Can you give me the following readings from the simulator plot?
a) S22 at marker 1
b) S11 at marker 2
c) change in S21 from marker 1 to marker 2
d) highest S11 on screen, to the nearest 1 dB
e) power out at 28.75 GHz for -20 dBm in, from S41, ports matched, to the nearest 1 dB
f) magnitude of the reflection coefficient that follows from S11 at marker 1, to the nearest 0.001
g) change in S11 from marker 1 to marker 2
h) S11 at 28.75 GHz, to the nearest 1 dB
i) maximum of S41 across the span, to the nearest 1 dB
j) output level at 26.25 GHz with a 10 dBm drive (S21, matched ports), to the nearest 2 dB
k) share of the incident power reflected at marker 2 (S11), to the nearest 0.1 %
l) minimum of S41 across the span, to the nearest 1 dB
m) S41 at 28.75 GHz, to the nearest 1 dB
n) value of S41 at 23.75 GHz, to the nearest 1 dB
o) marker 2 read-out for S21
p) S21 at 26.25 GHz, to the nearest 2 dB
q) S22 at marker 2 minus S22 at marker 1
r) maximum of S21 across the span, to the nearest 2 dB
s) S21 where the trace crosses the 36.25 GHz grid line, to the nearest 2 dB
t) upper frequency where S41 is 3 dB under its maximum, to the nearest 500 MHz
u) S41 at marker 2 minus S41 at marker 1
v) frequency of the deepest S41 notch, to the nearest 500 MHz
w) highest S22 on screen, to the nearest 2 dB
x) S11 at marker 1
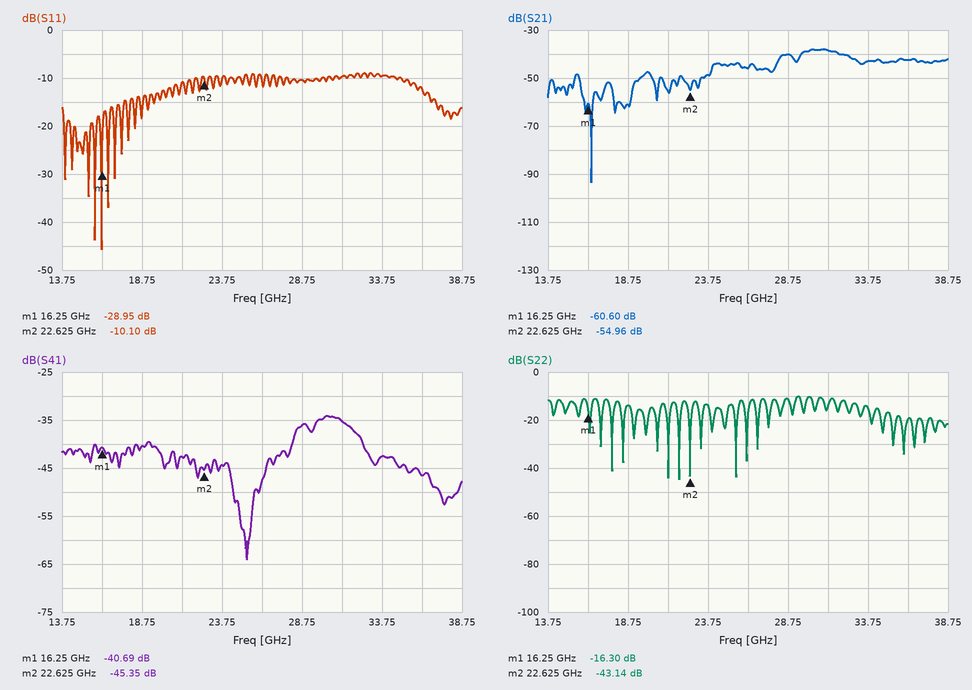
-16.30 dB
-10.10 dB
5.64 dB
-9 dB
-56 dBm
0.036
18.85 dB
-10 dB
-34 dB
-36 dBm
9.8 %
-64 dB
-36 dB
-44 dB
-54.96 dB
-46 dB
-26.84 dB
-38 dB
-42 dB
32.0 GHz
-4.66 dB
25.5 GHz
-10 dB
-28.95 dB
